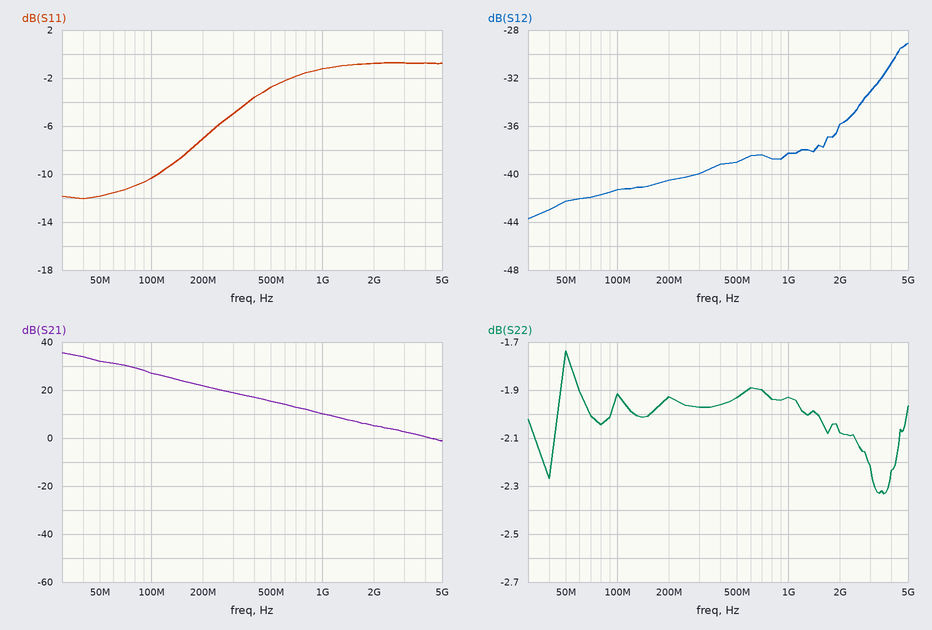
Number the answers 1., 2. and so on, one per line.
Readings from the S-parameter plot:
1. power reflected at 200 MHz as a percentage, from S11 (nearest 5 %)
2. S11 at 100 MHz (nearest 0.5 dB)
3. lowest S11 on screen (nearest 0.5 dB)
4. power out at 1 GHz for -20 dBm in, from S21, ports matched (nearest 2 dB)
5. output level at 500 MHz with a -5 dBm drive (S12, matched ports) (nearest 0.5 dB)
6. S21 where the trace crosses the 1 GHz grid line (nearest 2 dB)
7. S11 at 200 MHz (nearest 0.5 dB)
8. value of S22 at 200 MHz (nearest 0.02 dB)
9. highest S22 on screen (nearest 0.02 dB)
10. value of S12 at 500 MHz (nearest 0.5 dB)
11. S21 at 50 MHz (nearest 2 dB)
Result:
1. 20 %
2. -10.5 dB
3. -12.0 dB
4. -10 dBm
5. -44.0 dBm
6. 10 dB
7. -7.0 dB
8. -1.92 dB
9. -1.74 dB
10. -39.0 dB
11. 32 dB
